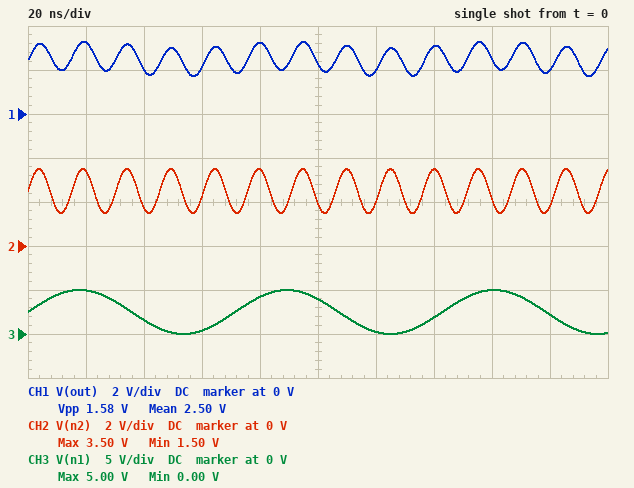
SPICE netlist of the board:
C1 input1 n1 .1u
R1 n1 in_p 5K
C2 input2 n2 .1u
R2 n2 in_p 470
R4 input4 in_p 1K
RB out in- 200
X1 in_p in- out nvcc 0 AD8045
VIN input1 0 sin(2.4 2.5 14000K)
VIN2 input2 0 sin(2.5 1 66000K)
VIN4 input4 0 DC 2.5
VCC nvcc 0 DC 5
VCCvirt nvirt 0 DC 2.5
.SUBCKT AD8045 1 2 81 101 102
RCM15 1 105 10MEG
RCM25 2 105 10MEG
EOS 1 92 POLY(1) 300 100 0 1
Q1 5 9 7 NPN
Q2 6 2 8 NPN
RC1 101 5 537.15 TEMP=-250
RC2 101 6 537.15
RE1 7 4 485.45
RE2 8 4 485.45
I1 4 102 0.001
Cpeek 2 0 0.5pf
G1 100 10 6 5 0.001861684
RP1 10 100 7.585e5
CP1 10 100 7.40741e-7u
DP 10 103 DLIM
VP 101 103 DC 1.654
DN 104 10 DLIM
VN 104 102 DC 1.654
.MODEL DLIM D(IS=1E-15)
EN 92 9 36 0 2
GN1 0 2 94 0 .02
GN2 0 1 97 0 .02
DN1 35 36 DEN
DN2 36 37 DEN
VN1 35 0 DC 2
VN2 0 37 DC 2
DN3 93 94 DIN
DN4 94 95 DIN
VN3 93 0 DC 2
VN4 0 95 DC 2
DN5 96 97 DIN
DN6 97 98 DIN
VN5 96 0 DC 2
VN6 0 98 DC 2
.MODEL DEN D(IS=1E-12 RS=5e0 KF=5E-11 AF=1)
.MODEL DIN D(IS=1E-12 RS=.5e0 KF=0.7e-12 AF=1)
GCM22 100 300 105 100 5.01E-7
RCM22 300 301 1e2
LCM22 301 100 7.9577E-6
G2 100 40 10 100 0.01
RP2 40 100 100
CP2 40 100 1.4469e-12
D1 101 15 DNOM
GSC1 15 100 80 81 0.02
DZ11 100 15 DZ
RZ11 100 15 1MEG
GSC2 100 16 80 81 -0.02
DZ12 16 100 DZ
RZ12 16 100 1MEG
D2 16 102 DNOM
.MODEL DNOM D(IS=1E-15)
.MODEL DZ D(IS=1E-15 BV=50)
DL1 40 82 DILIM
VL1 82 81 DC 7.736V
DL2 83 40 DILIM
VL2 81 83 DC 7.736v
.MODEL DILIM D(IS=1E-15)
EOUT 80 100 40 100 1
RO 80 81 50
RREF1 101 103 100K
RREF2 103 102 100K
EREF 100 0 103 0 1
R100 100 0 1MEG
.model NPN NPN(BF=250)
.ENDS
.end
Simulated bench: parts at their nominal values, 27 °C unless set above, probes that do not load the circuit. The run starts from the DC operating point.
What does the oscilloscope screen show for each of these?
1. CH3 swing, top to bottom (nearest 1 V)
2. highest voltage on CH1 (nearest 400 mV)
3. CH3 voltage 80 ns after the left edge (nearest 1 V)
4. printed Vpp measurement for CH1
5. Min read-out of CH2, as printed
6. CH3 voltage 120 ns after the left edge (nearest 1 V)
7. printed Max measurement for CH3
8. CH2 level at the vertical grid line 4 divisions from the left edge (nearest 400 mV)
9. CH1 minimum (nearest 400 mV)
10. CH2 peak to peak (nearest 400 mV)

5 V
3.2 V
4 V
1.58 V
1.50 V
0 V
5.00 V
3.6 V
1.6 V
2.0 V
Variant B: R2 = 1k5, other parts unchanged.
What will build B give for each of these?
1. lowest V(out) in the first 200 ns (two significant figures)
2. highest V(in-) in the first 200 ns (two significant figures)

1.9 V
3.1 V
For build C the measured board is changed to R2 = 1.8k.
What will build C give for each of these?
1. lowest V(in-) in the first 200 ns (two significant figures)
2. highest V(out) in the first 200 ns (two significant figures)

1.9 V
3.1 V
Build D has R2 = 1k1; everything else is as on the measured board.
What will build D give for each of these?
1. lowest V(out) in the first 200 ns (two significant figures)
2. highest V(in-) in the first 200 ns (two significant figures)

1.8 V
3.2 V
